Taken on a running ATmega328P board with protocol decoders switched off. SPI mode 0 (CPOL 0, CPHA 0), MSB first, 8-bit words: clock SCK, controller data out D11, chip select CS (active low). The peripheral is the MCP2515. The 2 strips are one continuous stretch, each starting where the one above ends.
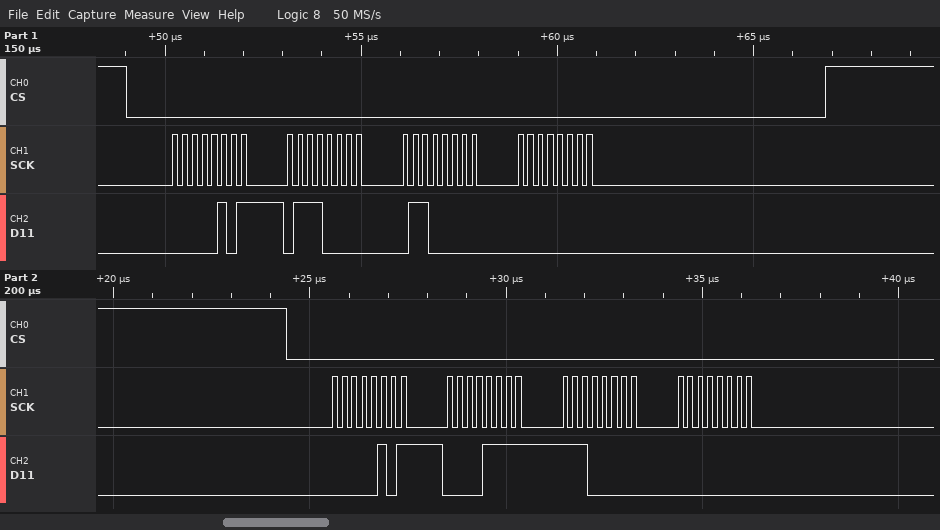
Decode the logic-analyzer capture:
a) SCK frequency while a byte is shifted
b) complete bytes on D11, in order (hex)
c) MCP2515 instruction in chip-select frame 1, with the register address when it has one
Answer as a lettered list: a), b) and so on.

a) 4 MHz
b) 05 70 60 00 05 0F E0 00
c) BIT MODIFY 0x70
